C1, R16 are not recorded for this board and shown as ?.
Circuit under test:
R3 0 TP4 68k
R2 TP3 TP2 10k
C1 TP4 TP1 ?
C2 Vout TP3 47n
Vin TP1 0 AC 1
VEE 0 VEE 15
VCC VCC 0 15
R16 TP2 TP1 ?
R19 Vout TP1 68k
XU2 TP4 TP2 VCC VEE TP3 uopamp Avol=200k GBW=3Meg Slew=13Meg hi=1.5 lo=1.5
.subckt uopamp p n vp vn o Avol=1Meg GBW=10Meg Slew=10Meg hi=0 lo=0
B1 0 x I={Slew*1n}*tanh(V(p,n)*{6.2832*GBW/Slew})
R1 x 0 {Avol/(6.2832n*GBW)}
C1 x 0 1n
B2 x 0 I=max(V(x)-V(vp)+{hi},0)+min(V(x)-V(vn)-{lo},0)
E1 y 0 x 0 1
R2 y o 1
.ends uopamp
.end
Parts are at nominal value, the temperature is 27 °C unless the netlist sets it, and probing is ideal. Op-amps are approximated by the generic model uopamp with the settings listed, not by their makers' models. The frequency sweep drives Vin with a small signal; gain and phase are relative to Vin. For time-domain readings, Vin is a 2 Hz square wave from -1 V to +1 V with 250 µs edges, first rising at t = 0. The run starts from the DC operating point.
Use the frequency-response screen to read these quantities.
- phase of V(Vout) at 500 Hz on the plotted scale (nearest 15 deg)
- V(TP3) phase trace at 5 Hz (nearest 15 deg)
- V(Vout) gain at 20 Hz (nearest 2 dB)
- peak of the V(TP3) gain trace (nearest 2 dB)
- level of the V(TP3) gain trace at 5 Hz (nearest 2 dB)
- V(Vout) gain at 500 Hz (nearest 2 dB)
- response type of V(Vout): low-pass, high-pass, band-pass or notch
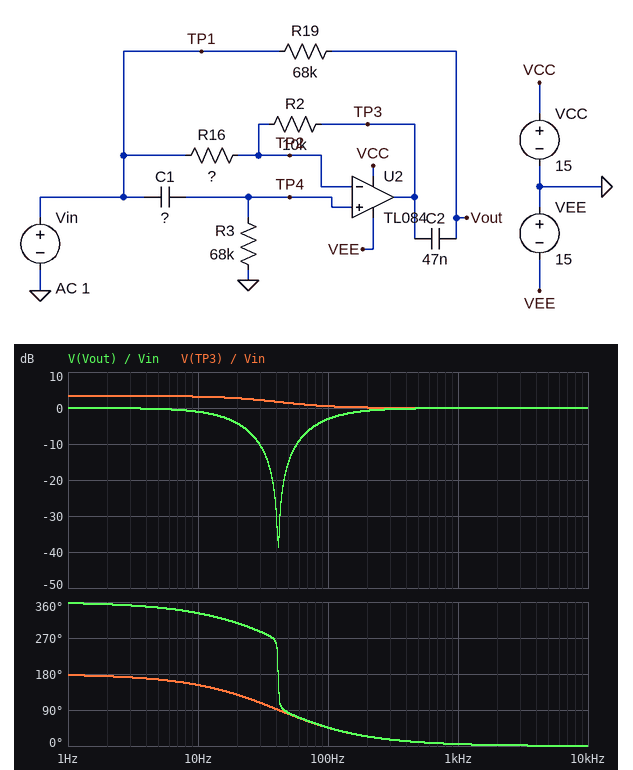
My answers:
15 deg
165 deg
-4 dB
4 dB
4 dB
0 dB
notch
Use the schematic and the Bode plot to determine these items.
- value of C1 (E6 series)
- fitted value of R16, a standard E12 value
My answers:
68 nF
6.8 kΩ
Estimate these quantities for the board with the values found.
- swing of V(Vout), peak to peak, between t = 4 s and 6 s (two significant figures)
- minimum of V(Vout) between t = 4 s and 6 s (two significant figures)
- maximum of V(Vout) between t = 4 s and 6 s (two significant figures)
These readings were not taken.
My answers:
2.0 V
-1.0 V
1.0 V
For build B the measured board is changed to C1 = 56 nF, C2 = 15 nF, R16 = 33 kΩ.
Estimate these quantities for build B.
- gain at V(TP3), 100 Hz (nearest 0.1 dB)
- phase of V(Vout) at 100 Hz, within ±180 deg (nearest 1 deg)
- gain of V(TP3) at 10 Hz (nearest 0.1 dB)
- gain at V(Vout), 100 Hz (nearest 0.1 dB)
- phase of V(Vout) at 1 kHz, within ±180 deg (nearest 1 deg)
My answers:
-0.6 dB
4 deg
-8.5 dB
-2.7 dB
3 deg
